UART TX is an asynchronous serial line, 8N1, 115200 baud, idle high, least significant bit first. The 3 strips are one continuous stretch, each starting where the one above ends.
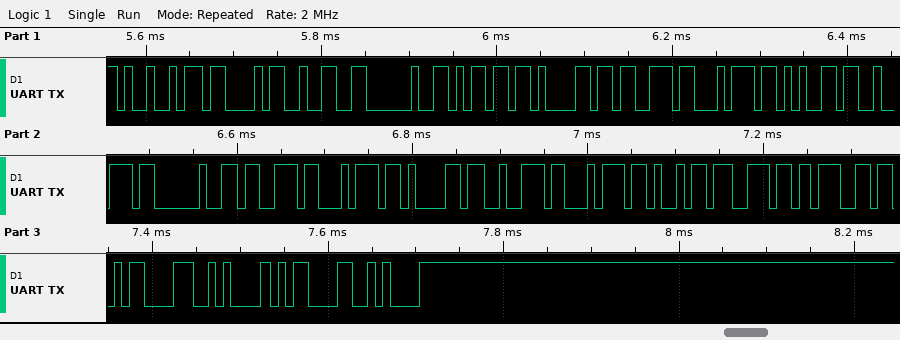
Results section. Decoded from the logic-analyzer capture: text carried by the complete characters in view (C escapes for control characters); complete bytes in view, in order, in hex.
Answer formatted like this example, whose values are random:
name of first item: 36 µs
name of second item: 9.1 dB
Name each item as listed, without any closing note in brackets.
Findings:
text carried by the complete characters in view: "IC2 master starting\r\n\r\n"
complete bytes in view, in order, in hex: 49 43 32 20 6D 61 73 74 65 72 20 73 74 61 72 74 69 6E 67 0D 0A 0D 0A
